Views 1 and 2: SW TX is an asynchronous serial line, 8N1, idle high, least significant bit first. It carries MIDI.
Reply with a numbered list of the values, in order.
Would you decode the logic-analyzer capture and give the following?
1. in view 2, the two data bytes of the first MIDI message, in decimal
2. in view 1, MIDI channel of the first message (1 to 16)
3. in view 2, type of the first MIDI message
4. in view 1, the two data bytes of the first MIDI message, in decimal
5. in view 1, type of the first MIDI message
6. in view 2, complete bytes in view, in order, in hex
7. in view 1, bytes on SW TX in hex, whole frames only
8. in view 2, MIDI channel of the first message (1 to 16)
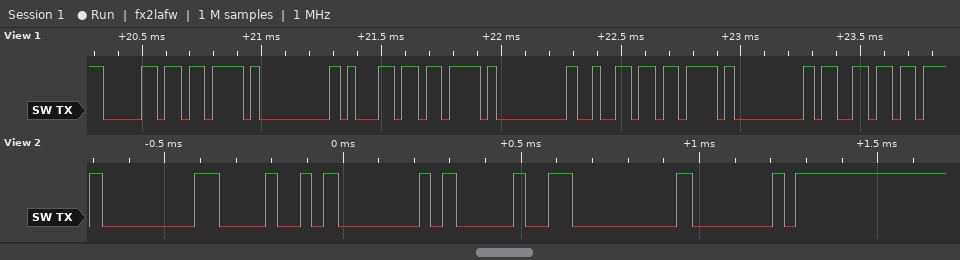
1. 72, 64
2. 1
3. Note Off
4. 123, 0
5. Control Change
6. 80 48 40 90 00 40
7. 0xB0 0x7B 0x00 0xB1 0x7B 0x00 0xB2 0x7B 0x00 0xB3
8. 1
